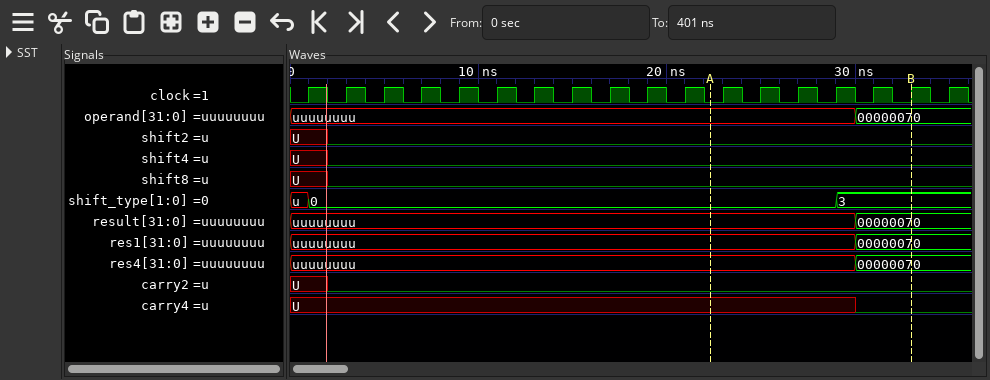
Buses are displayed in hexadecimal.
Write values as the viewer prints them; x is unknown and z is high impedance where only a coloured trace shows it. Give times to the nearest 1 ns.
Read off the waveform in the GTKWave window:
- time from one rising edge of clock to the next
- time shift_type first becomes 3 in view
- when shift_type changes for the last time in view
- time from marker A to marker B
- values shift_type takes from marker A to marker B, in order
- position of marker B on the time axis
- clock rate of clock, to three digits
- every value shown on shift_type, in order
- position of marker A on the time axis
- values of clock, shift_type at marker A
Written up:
2 ns
29 ns
29 ns
11 ns
0, 3
33 ns
500 MHz
u, 0, 3
22 ns
clock=0, shift_type=0
